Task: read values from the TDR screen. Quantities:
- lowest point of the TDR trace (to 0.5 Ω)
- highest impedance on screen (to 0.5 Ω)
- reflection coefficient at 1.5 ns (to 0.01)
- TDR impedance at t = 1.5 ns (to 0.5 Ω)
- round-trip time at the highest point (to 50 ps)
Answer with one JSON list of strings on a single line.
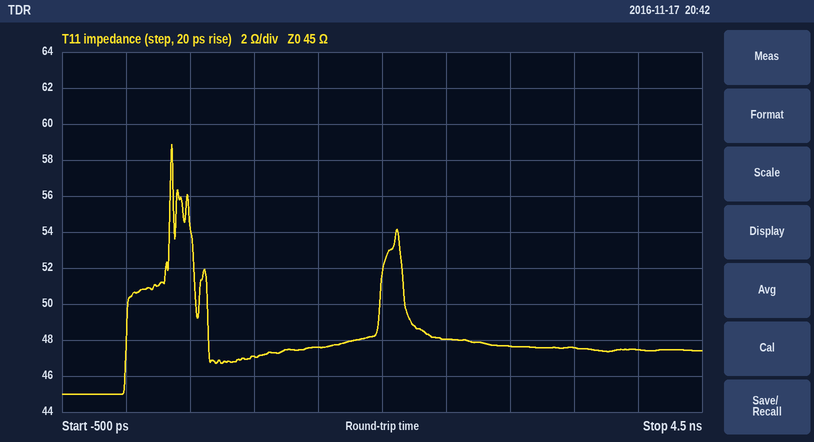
["45.0 Ω", "59.0 Ω", "+0.03", "47.5 Ω", "350 ps"]
